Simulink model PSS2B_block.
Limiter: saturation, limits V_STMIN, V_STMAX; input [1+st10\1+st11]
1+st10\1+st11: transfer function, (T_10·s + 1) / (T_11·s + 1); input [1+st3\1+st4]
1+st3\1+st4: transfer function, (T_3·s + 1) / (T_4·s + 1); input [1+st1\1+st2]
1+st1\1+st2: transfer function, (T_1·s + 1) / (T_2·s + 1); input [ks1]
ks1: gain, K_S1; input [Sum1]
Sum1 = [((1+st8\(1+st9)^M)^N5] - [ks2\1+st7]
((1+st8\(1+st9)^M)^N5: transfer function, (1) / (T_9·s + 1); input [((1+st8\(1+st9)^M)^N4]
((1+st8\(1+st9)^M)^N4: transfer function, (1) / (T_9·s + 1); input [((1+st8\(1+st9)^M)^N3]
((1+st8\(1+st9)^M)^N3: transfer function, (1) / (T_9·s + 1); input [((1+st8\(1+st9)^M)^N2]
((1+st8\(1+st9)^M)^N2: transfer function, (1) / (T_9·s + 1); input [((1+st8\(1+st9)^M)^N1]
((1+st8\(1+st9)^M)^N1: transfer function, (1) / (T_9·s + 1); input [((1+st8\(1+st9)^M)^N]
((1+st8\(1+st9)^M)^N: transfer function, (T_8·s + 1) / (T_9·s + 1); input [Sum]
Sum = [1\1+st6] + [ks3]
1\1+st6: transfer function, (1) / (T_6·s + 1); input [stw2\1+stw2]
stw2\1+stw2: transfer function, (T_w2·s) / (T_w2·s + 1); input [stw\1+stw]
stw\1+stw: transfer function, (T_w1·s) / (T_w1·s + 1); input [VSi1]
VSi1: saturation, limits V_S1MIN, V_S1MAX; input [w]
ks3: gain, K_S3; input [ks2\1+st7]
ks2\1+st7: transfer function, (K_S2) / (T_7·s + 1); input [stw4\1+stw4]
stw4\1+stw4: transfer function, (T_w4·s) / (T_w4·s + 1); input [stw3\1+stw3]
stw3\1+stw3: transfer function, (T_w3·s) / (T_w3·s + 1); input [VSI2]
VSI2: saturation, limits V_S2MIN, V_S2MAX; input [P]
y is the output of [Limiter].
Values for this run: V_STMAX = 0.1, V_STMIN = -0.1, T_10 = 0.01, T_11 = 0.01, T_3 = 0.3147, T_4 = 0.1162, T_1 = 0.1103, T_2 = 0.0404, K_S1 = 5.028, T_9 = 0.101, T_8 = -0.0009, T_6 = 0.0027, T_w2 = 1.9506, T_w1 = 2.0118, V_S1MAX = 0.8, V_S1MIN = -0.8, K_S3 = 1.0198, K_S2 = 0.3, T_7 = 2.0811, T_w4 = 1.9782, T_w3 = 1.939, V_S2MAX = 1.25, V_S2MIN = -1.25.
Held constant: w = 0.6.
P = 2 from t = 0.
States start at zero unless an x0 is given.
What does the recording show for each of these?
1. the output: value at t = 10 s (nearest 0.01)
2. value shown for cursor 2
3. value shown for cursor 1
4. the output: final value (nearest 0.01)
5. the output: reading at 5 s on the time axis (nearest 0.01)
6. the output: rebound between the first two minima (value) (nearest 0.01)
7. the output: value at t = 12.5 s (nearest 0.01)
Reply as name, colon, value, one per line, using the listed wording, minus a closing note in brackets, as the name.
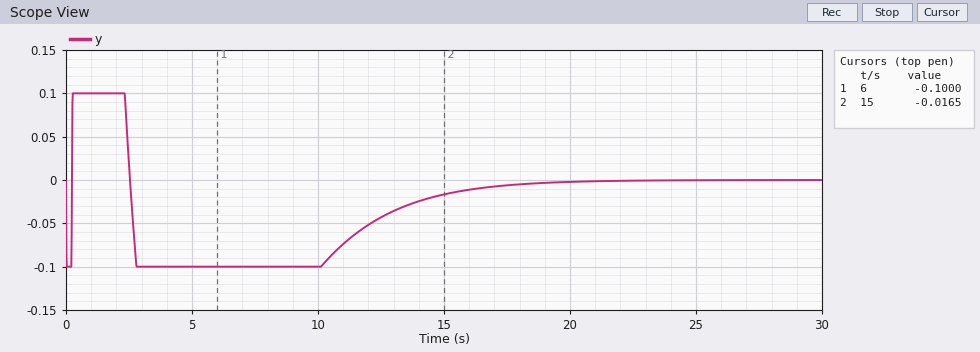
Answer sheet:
the output: value at t = 10 s: -0.10
value shown for cursor 2: -0.0165
value shown for cursor 1: -0.1000
the output: final value: 0.00
the output: reading at 5 s on the time axis: -0.10
the output: rebound between the first two minima (value): 0.10
the output: value at t = 12.5 s: -0.04
